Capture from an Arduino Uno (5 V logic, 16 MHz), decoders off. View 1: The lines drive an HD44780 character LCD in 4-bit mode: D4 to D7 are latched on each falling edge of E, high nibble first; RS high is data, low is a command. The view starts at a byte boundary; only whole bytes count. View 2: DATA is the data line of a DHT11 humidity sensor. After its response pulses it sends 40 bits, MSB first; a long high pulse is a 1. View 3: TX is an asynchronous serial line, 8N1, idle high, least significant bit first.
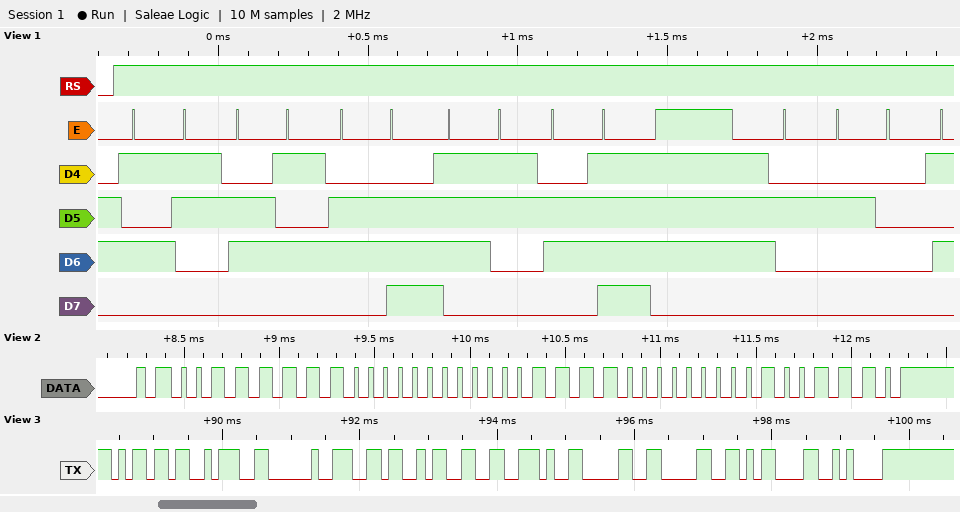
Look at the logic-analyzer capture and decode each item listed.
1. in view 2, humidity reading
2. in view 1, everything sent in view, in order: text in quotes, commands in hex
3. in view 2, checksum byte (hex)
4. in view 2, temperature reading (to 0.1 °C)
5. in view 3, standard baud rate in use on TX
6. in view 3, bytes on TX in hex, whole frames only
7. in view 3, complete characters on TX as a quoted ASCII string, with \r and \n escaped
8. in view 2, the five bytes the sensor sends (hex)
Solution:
63 %
"Sensor "
0x4E
15.0 °C
9600 baud
0x6D 0x3A 0x20 0x36 0x33 0x2E 0x30 0x30 0x0D 0x0A
"m: 63.00\r\n"
3F 00 0F 00 4E
